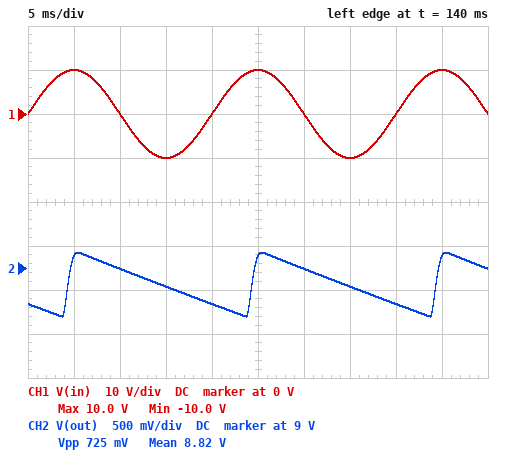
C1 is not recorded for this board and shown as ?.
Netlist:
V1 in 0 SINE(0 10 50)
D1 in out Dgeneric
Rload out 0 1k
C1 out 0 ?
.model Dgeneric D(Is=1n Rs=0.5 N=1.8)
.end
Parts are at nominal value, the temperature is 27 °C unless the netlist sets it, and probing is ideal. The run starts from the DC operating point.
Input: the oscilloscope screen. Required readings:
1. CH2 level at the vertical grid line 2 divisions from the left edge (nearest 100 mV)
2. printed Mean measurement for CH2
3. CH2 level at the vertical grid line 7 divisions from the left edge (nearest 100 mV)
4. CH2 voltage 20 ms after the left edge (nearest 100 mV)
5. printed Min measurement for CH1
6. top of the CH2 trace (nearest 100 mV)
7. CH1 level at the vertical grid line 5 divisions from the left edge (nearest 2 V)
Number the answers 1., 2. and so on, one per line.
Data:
1. 9.0 V
2. 8.82 V
3. 8.8 V
4. 8.6 V
5. -10.0 V
6. 9.2 V
7. 10 V
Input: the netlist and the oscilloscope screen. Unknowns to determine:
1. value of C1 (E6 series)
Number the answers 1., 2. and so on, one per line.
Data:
1. 220 µF
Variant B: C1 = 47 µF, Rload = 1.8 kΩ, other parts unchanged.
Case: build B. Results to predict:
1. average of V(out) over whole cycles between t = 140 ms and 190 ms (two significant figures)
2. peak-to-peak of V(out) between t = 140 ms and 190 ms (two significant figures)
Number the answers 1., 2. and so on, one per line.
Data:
1. 8.4 V
2. 1.7 V
